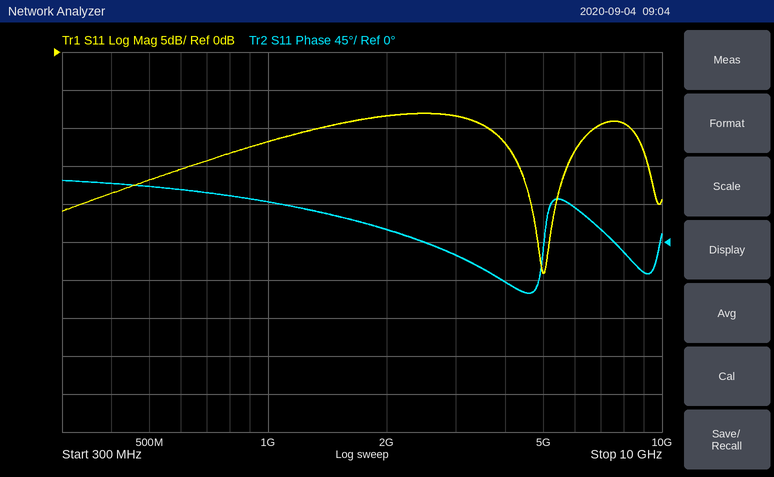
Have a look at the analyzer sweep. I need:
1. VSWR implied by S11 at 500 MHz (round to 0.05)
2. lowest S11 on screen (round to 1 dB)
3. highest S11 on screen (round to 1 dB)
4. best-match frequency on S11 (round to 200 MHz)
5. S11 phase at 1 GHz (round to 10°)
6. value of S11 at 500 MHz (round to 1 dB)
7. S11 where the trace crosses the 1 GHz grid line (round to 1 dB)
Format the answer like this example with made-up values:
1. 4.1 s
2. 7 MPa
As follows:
1. 1.35
2. -29 dB
3. -8 dB
4. 5.0 GHz
5. 50°
6. -17 dB
7. -12 dB
